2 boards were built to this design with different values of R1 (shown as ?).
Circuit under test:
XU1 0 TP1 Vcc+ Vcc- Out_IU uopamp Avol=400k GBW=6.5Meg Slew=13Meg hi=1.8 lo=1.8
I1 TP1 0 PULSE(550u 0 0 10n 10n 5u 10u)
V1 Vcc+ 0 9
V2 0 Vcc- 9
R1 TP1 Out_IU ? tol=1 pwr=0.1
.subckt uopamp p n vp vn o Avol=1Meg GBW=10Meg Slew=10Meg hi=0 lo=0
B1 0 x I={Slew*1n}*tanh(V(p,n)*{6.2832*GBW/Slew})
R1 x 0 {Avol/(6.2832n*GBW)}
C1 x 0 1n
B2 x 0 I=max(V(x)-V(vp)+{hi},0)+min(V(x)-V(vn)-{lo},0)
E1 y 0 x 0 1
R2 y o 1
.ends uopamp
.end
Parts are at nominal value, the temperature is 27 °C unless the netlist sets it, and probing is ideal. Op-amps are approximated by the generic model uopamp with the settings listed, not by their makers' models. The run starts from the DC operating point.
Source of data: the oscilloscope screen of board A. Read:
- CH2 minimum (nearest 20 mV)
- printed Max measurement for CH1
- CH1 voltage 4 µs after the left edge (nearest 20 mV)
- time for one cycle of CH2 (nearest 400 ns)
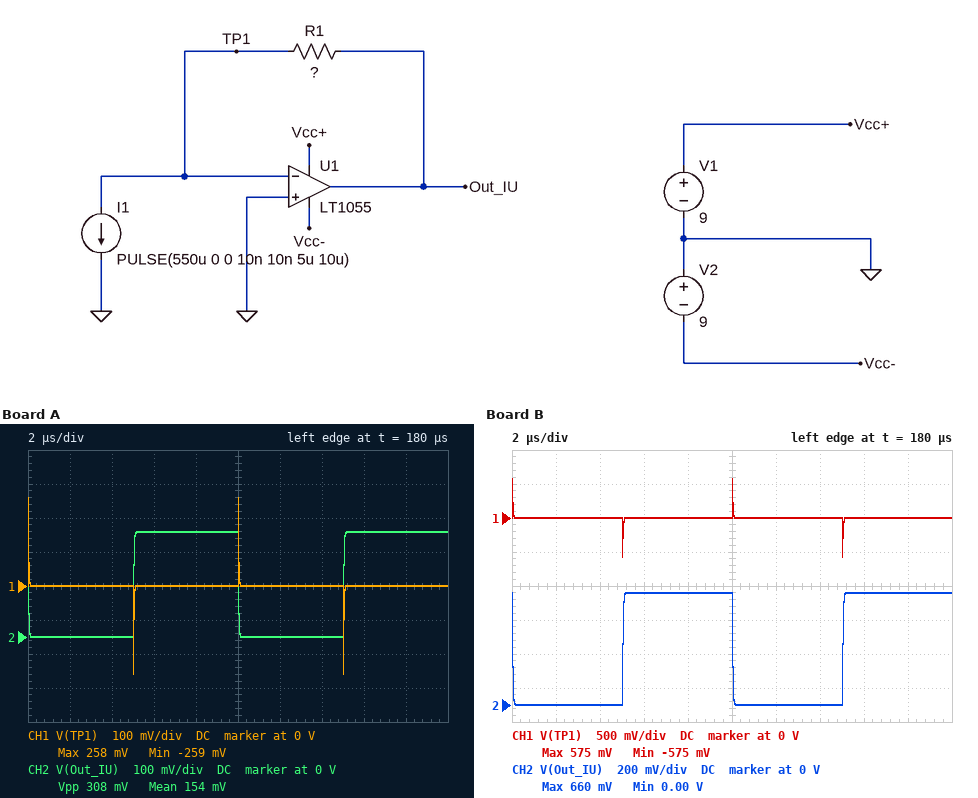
0 V
258 mV
0 V
10.0 µs
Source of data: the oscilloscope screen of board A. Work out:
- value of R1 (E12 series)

560 Ω
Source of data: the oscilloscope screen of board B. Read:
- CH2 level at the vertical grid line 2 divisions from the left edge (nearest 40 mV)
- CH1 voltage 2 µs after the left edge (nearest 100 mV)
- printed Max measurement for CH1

0 V
0 V
575 mV
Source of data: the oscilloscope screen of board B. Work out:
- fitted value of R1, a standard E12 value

1.2 kΩ
